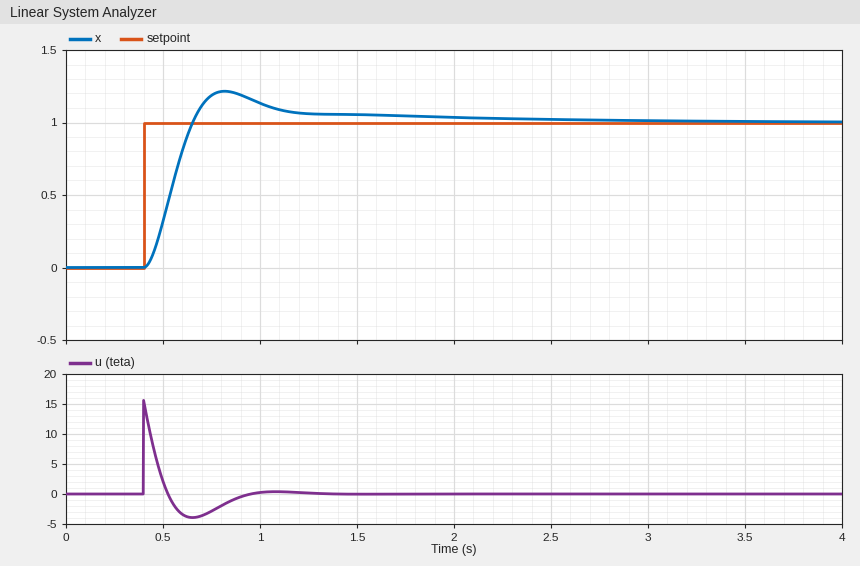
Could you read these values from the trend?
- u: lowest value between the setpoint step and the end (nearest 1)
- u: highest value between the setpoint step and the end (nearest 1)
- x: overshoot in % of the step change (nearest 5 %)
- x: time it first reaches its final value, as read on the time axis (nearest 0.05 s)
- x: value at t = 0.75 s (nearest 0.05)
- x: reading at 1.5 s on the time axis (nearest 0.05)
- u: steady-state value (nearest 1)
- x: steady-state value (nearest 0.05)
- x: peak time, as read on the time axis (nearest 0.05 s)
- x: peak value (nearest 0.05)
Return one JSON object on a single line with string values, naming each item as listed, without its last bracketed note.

{"u: lowest value between the setpoint step and the end": "-4", "u: highest value between the setpoint step and the end": "16", "x: overshoot in % of the step change": "20 %", "x: time it first reaches its final value, as read on the time axis": "0.65 s", "x: value at t = 0.75 s": "1.20", "x: reading at 1.5 s on the time axis": "1.05", "u: steady-state value": "0", "x: steady-state value": "1.00", "x: peak time, as read on the time axis": "0.80 s", "x: peak value": "1.20"}
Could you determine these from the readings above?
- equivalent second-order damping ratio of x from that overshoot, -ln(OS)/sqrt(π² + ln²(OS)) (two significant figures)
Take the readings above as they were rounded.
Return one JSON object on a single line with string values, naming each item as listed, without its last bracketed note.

{"equivalent second-order damping ratio of x from that overshoot, -ln(OS)/sqrt(π² + ln²(OS))": "0.46"}
